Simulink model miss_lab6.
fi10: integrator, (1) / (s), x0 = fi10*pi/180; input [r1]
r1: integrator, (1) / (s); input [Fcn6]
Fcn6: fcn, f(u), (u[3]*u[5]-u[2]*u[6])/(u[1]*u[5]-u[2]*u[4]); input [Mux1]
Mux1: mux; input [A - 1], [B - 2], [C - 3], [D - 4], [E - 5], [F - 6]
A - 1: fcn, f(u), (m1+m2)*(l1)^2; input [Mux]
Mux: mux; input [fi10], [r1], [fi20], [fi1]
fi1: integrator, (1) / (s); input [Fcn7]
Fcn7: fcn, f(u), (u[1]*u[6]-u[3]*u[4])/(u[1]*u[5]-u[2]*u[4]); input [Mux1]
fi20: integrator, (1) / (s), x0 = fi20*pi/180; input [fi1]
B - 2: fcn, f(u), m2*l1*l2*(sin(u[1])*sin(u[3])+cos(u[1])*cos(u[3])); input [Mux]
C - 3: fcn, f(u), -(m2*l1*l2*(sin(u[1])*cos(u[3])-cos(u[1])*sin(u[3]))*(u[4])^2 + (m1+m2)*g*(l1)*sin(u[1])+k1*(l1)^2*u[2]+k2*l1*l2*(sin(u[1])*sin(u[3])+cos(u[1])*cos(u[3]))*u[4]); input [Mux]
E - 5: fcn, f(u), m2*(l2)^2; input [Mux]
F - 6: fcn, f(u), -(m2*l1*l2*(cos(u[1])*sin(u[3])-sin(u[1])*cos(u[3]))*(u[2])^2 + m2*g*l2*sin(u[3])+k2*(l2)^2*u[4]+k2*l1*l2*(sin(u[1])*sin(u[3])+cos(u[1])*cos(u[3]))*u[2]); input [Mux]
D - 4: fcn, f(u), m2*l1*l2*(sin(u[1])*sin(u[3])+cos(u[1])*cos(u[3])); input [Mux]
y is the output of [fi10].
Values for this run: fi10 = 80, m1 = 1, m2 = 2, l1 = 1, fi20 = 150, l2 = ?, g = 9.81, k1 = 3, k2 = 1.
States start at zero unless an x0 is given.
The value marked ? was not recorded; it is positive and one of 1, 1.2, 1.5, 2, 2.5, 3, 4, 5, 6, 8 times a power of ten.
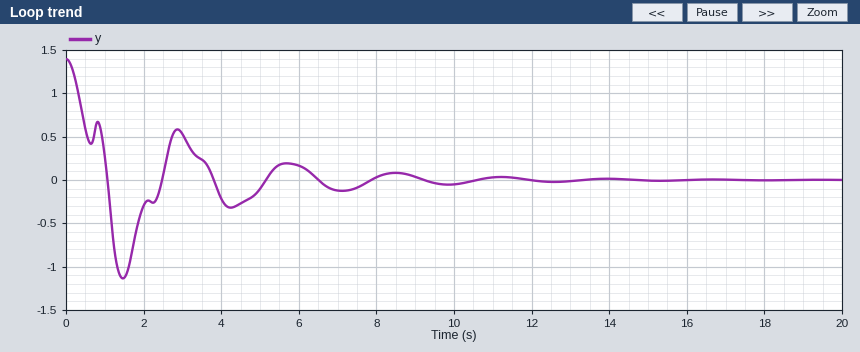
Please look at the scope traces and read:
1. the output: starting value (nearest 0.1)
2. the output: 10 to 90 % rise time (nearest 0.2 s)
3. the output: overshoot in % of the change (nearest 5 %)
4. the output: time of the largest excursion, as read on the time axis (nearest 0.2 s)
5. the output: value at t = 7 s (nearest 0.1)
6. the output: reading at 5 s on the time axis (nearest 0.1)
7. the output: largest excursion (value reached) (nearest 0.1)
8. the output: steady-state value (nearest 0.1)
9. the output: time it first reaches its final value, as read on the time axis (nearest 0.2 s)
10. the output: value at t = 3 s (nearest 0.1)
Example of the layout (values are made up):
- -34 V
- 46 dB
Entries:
- 1.4
- 0.8 s
- 80 %
- 1.4 s
- -0.1
- -0.1
- -1.1
- 0.0
- 1.0 s
- 0.5
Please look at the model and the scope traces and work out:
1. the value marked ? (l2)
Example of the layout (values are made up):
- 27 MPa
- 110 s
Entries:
- 1
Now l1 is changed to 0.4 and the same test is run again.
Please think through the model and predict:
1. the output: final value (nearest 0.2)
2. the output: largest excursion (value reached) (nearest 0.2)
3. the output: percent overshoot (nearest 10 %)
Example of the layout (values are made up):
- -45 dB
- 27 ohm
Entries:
- 0.0
- -1.8
- 130 %
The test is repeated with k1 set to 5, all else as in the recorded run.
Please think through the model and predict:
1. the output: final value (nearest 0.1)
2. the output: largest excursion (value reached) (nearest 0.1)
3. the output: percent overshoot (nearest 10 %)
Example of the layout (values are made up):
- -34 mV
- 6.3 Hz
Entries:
- 0.0
- -0.8
- 60 %
